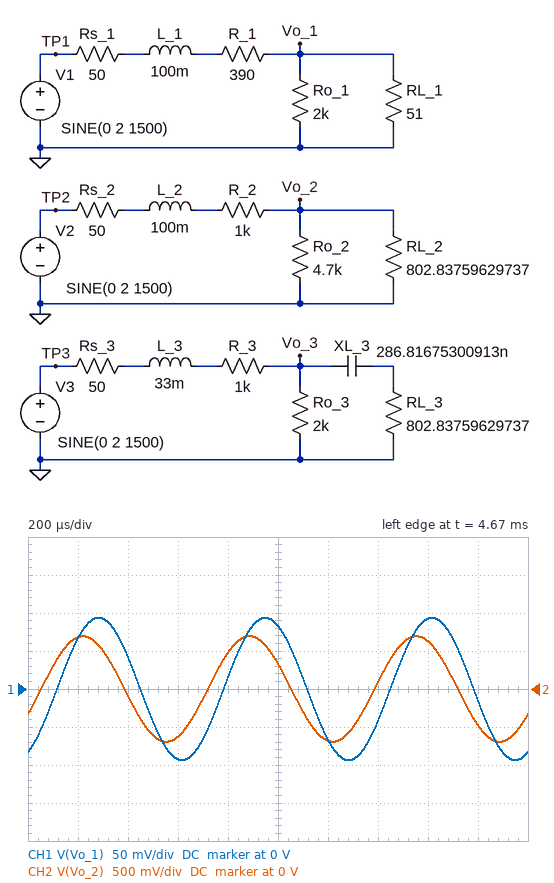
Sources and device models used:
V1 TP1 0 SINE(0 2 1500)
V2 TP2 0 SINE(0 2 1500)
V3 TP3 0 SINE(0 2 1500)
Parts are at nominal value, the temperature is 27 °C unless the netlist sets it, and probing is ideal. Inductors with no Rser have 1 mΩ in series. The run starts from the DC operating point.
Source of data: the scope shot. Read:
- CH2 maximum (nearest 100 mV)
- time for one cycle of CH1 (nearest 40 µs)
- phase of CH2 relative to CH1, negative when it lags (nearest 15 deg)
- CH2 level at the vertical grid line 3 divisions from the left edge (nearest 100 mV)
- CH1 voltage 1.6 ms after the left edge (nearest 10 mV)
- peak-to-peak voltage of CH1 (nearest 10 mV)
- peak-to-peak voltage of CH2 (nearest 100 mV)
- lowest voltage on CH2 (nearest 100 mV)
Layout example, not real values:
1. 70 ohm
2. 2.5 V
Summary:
1. 700 mV
2. 680 µs
3. 30 deg
4. -600 mV
5. 90 mV
6. 190 mV
7. 1.4 V
8. -700 mV
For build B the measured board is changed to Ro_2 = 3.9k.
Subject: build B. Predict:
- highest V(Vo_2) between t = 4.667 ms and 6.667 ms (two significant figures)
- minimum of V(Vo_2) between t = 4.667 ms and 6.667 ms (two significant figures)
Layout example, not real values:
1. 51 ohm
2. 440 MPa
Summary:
1. 680 mV
2. -680 mV
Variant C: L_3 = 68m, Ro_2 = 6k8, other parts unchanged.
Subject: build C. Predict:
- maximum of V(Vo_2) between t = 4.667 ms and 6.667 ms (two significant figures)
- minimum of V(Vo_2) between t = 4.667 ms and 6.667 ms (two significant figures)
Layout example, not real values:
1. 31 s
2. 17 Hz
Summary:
1. 720 mV
2. -720 mV
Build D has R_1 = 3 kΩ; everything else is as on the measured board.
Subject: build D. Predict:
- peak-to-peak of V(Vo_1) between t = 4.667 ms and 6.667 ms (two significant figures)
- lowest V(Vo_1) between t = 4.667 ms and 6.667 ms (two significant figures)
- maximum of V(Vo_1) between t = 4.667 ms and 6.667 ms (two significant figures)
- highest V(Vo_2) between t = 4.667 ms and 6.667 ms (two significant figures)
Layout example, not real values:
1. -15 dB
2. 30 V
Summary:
1. 61 mV
2. -31 mV
3. 31 mV
4. 690 mV
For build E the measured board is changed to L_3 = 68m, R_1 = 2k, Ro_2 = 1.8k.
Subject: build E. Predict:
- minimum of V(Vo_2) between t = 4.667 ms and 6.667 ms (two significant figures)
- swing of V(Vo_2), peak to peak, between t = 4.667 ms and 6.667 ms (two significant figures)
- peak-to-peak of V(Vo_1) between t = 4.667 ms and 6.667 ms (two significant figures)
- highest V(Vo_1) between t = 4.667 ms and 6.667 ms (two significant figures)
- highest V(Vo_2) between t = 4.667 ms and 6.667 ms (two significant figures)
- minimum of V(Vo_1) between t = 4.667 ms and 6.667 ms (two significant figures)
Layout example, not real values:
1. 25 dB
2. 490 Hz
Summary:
1. -600 mV
2. 1.2 V
3. 86 mV
4. 43 mV
5. 600 mV
6. -43 mV
